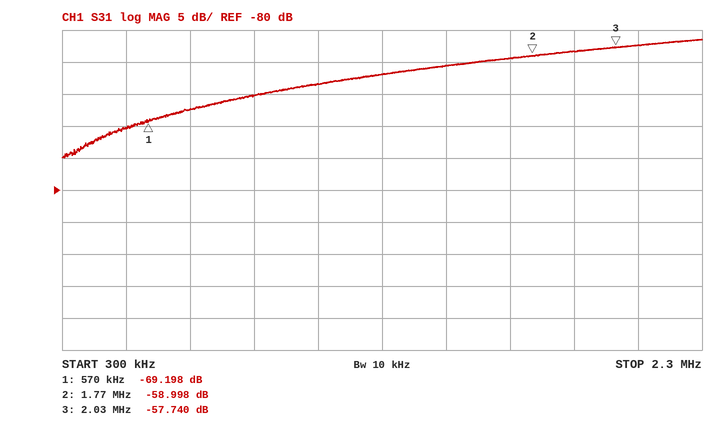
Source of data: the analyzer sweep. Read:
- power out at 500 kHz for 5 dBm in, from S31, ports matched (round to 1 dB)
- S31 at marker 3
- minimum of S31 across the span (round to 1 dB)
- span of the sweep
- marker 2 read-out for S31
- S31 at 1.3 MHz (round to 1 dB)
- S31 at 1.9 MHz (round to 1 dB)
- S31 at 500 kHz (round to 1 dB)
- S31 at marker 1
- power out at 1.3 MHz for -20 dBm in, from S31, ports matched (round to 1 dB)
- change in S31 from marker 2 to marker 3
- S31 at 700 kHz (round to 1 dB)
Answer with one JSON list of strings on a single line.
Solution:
["-65 dBm", "-57.740 dB", "-75 dB", "2 MHz", "-58.998 dB", "-62 dB", "-58 dB", "-70 dB", "-69.198 dB", "-82 dBm", "1.258 dB", "-67 dB"]
